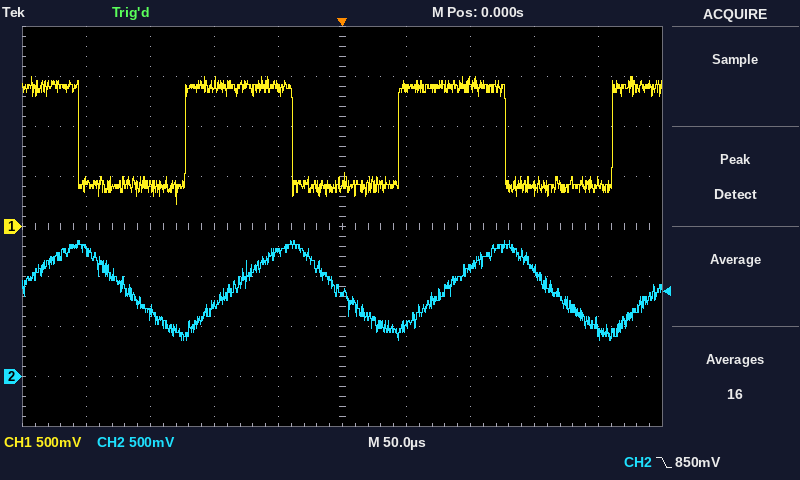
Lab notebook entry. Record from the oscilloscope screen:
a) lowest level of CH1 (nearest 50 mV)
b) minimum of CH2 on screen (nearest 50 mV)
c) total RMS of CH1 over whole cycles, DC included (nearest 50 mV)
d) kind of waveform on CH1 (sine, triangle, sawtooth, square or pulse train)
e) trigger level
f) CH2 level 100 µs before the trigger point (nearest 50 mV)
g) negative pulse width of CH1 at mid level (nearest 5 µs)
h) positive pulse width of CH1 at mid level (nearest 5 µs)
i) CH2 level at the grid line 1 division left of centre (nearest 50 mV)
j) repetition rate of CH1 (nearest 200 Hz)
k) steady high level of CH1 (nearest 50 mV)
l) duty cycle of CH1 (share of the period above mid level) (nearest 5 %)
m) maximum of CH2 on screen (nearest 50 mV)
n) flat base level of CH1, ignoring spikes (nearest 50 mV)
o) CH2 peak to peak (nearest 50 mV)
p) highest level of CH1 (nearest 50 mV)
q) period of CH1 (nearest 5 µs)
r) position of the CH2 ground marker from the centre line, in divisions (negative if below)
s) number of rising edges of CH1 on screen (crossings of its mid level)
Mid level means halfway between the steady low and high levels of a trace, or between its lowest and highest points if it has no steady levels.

200 mV
350 mV
1.05 V
square
850 mV
700 mV
85 µs
85 µs
1.25 V
6.0 kHz
1.40 V
50 %
1.35 V
400 mV
1.00 V
1.50 V
165 µs
-3.0 div
3
